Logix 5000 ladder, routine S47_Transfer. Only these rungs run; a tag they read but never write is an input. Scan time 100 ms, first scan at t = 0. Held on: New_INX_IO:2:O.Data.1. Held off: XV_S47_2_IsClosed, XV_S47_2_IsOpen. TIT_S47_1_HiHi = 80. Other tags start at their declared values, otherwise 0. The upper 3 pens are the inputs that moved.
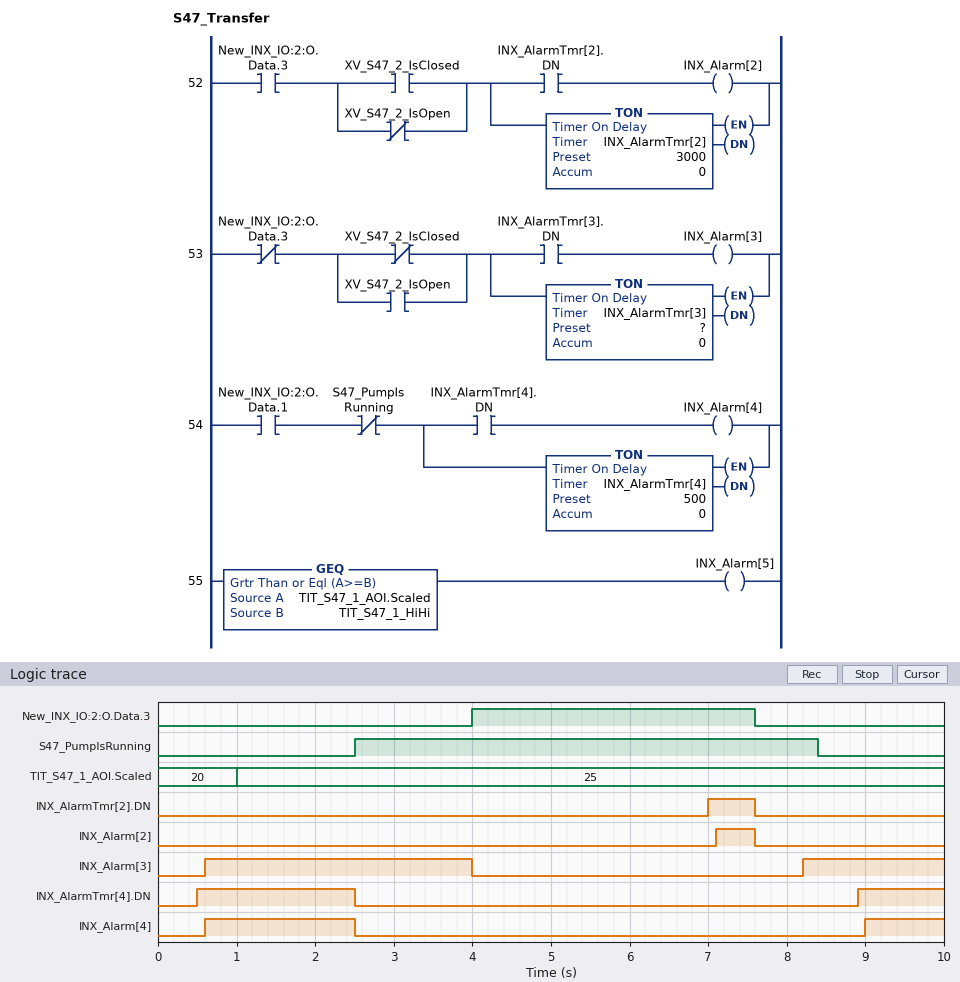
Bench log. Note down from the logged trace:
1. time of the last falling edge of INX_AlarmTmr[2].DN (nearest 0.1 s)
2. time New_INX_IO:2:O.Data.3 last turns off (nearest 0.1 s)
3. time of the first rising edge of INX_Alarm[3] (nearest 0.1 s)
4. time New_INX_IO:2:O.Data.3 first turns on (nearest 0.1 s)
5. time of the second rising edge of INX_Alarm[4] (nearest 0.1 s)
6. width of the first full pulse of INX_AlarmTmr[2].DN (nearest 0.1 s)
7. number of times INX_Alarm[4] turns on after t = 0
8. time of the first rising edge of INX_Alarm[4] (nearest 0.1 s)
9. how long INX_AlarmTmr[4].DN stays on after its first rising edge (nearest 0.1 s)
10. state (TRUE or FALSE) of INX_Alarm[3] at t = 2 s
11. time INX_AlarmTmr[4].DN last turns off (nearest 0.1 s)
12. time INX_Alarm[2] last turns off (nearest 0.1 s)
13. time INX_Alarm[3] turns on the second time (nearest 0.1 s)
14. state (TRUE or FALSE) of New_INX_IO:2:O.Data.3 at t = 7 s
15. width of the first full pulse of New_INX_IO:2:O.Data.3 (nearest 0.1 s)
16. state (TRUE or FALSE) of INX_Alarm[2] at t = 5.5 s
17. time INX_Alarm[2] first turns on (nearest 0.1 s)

7.6 s
7.6 s
0.6 s
4.0 s
9.0 s
0.6 s
2
0.6 s
2.0 s
TRUE
2.5 s
7.6 s
8.2 s
TRUE
3.6 s
FALSE
7.1 s
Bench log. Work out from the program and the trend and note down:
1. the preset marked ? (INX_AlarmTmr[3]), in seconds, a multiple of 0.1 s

0.5 s
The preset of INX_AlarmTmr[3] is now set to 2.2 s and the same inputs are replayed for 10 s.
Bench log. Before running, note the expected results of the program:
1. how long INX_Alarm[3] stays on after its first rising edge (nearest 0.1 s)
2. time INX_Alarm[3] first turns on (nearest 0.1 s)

1.7 s
2.3 s
